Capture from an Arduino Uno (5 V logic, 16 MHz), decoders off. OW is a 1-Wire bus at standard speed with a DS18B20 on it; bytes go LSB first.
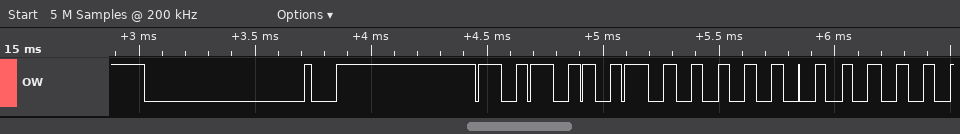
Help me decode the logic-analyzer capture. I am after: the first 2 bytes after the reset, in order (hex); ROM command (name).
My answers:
55 00
Match ROM
